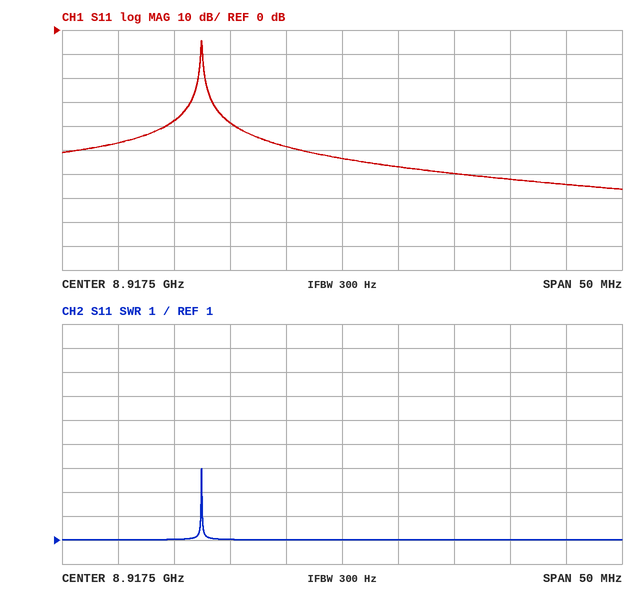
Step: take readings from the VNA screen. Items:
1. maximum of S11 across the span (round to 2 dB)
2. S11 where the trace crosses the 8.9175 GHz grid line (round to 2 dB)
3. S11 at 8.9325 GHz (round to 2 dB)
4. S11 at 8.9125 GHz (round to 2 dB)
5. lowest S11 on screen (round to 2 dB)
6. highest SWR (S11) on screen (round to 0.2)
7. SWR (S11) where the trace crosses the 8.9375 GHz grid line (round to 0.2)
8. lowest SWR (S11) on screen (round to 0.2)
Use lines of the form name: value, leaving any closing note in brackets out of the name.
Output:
maximum of S11 across the span: -4 dB
S11 where the trace crosses the 8.9175 GHz grid line: -54 dB
S11 at 8.9325 GHz: -62 dB
S11 at 8.9125 GHz: -48 dB
lowest S11 on screen: -66 dB
highest SWR (S11) on screen: 4.0
SWR (S11) where the trace crosses the 8.9375 GHz grid line: 1.0
lowest SWR (S11) on screen: 1.0
